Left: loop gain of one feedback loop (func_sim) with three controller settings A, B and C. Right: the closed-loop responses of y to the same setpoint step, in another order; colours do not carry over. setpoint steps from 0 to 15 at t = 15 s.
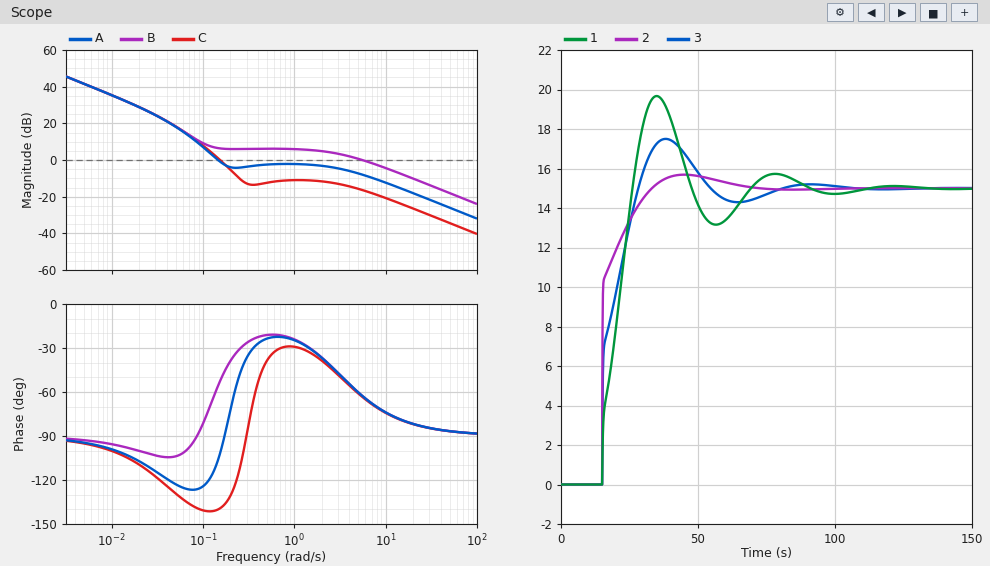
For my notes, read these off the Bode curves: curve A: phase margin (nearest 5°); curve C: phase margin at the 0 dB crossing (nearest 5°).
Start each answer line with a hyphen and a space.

- 75°
- 40°
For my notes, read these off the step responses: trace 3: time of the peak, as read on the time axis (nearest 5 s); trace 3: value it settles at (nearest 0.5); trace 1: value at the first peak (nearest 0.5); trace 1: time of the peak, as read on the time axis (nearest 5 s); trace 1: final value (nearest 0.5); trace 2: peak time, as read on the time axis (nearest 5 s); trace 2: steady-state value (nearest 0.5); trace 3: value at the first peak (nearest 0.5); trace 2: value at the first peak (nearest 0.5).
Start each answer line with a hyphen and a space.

- 40 s
- 15.0
- 19.5
- 35 s
- 15.0
- 45 s
- 15.0
- 17.5
- 15.5
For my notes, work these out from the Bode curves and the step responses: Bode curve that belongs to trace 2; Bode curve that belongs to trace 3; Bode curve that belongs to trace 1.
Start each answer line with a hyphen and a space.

- B
- A
- C
